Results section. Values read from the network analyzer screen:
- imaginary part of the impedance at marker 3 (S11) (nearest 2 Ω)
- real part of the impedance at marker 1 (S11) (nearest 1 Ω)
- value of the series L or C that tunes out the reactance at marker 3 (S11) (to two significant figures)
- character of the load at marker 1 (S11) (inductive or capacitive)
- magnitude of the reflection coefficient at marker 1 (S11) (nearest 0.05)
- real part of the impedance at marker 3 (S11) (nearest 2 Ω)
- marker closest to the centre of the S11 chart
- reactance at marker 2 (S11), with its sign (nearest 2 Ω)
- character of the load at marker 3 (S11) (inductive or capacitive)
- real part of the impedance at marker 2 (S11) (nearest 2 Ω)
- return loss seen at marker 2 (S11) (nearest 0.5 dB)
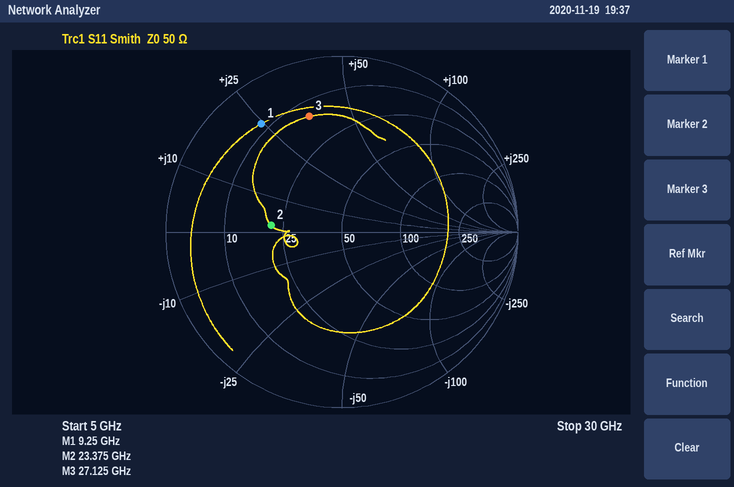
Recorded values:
+36 Ω
8 Ω
160 fF
inductive
0.75
14 Ω
marker 2
+2 Ω
inductive
22 Ω
8.0 dB
